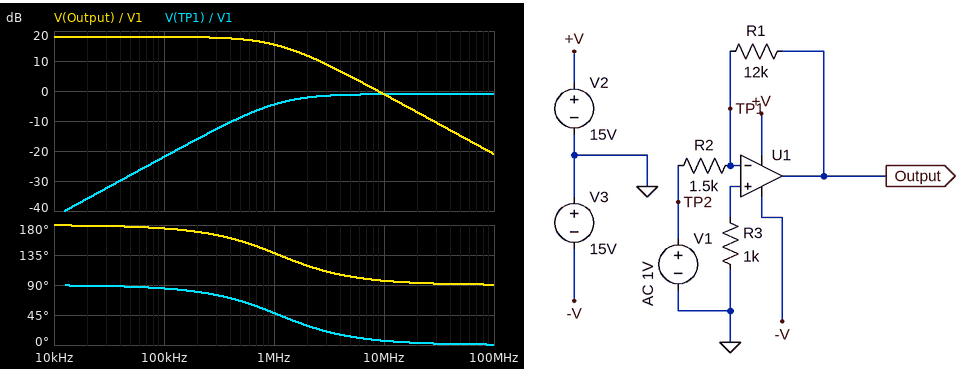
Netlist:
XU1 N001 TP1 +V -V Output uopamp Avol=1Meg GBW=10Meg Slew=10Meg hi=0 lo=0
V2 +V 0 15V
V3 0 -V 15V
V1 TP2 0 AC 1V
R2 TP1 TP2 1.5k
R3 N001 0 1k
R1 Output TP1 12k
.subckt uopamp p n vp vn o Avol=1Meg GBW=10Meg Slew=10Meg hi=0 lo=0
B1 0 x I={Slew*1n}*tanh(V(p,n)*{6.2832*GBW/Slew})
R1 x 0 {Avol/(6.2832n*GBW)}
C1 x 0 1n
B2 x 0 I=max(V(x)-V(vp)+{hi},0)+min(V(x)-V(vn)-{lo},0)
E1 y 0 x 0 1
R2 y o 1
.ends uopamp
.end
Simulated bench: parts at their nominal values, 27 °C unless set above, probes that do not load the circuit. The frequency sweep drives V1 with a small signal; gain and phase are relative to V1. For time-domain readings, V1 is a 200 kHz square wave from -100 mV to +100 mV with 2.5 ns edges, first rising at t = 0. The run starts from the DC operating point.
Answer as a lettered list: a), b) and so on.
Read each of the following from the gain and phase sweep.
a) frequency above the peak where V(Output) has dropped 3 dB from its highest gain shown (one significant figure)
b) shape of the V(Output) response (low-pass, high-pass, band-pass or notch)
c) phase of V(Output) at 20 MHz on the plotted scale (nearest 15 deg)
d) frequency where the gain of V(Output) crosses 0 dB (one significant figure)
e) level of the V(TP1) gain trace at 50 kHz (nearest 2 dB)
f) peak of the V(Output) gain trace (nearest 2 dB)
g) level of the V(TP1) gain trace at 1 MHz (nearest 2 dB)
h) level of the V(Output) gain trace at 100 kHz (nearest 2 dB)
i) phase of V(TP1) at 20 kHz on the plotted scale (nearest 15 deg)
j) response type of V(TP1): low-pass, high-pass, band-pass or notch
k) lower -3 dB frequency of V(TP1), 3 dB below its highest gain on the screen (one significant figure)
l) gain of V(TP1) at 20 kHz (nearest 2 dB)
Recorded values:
a) 1 MHz
b) low-pass
c) 90 deg
d) 9 MHz
e) -28 dB
f) 18 dB
g) -4 dB
h) 18 dB
i) 90 deg
j) high-pass
k) 1 MHz
l) -36 dB
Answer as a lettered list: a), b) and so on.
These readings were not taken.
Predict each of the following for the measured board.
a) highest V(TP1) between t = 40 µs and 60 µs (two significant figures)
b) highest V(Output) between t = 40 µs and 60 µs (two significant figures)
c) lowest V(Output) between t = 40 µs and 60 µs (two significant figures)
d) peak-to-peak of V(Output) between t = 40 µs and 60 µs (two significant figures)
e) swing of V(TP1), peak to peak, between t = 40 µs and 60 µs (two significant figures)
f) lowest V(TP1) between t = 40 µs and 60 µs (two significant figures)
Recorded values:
a) 180 mV
b) 800 mV
c) -800 mV
d) 1.6 V
e) 350 mV
f) -180 mV
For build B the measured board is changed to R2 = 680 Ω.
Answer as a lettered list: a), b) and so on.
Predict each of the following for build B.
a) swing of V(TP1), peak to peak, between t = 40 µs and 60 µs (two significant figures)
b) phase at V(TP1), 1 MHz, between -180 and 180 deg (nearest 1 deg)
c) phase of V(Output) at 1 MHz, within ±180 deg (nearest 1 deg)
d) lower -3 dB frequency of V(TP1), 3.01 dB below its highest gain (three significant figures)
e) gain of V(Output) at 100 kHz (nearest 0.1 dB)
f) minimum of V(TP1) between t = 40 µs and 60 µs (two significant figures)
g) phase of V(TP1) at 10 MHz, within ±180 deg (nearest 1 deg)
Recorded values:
a) 380 mV
b) 28 deg
c) 118 deg
d) 536 kHz
e) 24.8 dB
f) -190 mV
g) 3 deg
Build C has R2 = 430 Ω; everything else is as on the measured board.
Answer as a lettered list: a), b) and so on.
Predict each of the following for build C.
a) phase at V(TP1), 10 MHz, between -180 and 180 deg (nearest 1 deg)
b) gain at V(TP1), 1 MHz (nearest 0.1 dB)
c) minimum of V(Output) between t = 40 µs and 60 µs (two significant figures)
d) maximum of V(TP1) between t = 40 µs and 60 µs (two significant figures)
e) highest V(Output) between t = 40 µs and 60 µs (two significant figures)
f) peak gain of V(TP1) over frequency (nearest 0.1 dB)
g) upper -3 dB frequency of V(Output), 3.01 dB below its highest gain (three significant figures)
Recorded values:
a) 2 deg
b) -0.8 dB
c) -2.8 V
d) 190 mV
e) 2.8 V
f) -0.3 dB
g) 346 kHz
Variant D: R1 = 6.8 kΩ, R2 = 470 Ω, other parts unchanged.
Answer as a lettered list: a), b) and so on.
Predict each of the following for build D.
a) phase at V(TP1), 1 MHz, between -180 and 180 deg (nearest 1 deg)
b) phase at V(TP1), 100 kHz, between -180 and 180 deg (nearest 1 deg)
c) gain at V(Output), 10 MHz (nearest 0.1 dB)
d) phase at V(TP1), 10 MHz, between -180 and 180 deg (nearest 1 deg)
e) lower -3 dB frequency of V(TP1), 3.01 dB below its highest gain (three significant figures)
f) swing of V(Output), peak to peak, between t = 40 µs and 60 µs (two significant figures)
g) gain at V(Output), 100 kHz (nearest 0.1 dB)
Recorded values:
a) 33 deg
b) 81 deg
c) -0.6 dB
d) 4 deg
e) 646 kHz
f) 2.9 V
g) 23.1 dB
